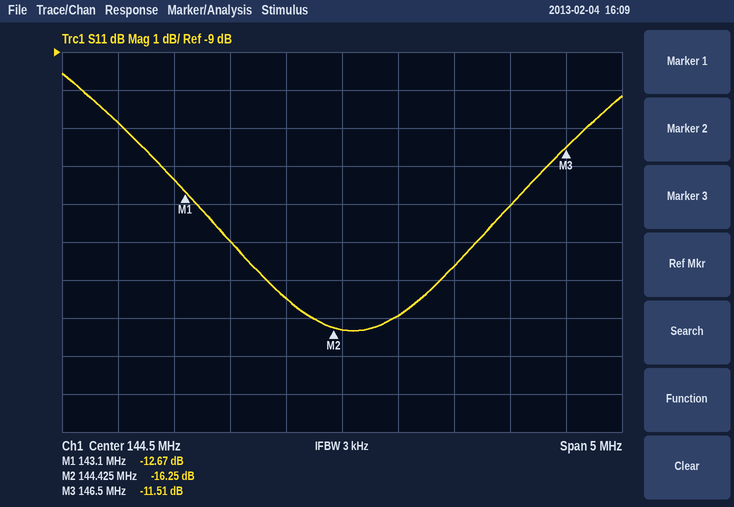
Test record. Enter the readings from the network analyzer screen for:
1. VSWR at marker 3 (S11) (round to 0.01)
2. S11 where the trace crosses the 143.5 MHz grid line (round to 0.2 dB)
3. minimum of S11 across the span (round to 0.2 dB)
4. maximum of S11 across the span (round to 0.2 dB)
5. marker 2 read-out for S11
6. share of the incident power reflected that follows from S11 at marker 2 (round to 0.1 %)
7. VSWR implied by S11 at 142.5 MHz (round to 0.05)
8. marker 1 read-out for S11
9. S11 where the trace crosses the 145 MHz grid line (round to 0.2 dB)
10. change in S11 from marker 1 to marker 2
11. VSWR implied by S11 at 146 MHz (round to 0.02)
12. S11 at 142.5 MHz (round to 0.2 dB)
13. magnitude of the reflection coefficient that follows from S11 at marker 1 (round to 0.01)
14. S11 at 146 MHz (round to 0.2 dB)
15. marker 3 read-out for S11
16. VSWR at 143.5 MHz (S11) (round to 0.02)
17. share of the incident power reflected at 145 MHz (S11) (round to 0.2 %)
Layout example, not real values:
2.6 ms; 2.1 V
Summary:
1.72; -14.0 dB; -16.4 dB; -9.6 dB; -16.25 dB; 2.4 %; 1.80; -12.67 dB; -16.0 dB; -3.58 dB; 1.58; -10.8 dB; 0.23; -13.0 dB; -11.51 dB; 1.50; 2.6 %
